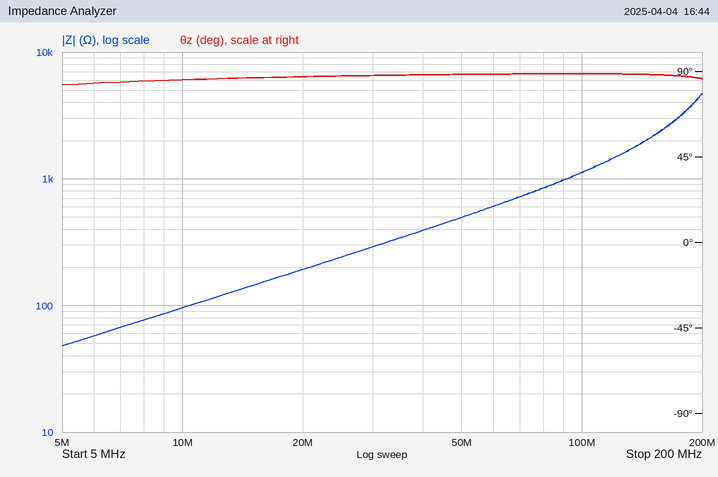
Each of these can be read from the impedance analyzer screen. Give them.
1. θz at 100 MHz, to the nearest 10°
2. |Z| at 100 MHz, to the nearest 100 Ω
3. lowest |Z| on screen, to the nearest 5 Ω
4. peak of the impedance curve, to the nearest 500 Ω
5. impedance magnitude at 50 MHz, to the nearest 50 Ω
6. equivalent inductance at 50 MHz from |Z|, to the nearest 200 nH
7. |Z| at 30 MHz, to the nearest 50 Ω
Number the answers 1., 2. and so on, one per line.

1. 90°
2. 1.1 kΩ
3. 50 Ω
4. 4.5 kΩ
5. 500 Ω
6. 1.6 µH
7. 300 Ω
